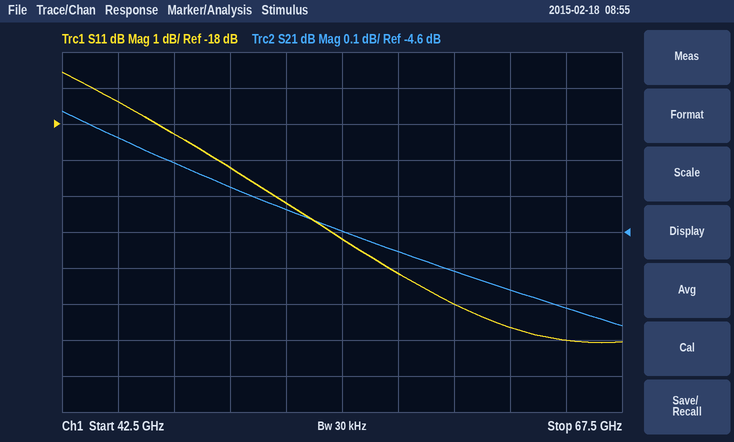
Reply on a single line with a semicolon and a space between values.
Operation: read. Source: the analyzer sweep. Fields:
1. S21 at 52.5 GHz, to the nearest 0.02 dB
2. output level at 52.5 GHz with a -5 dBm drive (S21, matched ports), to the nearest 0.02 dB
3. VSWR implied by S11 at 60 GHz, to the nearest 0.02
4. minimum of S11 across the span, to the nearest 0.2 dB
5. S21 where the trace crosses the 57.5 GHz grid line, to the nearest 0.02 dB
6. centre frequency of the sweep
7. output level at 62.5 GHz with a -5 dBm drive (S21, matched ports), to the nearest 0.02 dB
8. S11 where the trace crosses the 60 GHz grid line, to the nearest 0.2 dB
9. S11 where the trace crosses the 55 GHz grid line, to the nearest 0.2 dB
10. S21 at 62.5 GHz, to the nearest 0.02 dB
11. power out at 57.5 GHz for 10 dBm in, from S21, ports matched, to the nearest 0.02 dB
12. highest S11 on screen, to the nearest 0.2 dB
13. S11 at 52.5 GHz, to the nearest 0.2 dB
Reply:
-4.54 dB; -9.54 dBm; 1.16; -24.0 dB; -4.66 dB; 55 GHz; -9.76 dBm; -23.0 dB; -21.2 dB; -4.76 dB; 5.34 dBm; -16.6 dB; -20.2 dB
